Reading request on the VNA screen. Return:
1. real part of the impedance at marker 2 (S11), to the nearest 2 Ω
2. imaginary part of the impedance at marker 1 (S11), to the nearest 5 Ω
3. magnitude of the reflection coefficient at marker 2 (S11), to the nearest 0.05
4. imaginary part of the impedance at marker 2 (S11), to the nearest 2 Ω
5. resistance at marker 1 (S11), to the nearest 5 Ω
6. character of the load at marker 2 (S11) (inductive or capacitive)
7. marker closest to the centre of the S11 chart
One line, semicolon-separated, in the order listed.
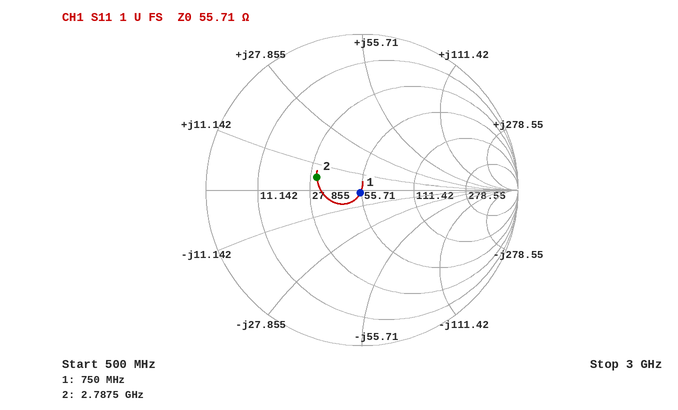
30 Ω; 0 Ω; 0.30; +6 Ω; 55 Ω; inductive; marker 1
